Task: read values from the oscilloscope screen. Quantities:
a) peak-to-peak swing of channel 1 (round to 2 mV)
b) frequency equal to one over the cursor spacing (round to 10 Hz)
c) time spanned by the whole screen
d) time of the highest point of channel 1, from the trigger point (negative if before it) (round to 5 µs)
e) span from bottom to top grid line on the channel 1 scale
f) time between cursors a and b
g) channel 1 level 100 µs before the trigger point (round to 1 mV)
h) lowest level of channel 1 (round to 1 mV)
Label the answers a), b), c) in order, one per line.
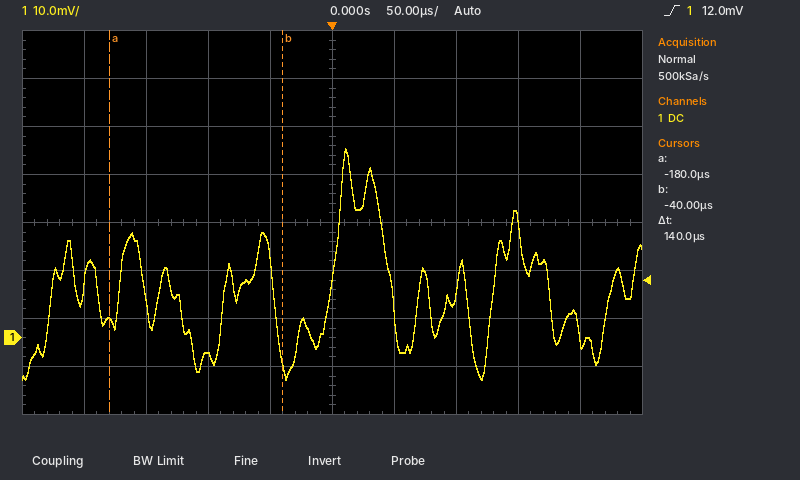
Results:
a) 48 mV
b) 7.14 kHz
c) 500 µs
d) +10 µs
e) 80 mV
f) 140 µs
g) -4 mV
h) -9 mV
